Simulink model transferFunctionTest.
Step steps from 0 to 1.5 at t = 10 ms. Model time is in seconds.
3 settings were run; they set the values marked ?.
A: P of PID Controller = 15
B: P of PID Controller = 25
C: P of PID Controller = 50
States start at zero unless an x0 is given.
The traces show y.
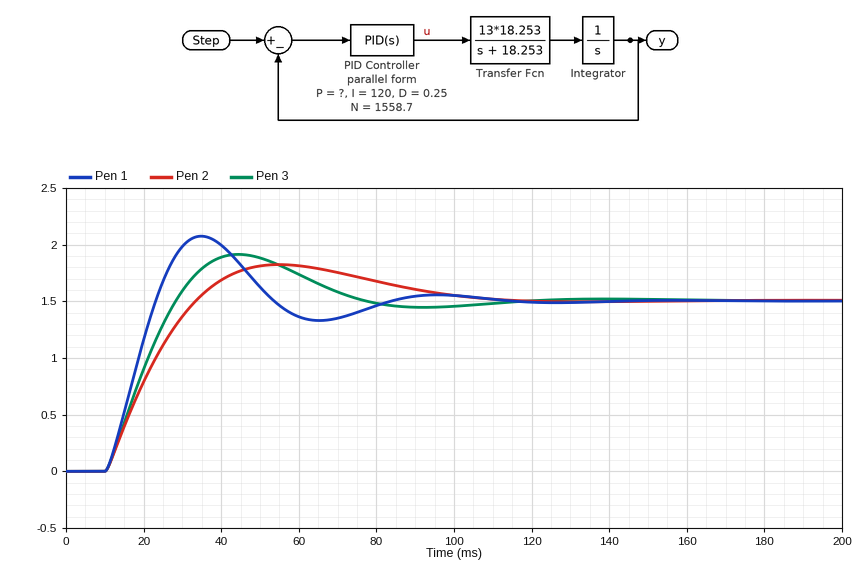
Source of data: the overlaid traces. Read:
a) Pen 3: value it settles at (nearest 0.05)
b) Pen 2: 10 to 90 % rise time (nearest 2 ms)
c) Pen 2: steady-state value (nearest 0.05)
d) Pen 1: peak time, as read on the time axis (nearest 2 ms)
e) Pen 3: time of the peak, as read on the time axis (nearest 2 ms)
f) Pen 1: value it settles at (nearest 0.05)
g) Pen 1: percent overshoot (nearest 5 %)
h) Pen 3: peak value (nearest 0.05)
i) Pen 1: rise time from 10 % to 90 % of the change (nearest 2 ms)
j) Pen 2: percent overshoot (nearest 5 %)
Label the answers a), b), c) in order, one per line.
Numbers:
a) 1.50
b) 18 ms
c) 1.50
d) 34 ms
e) 44 ms
f) 1.50
g) 40 %
h) 1.90
i) 10 ms
j) 20 %
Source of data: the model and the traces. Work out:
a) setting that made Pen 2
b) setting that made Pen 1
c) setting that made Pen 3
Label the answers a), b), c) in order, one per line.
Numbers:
a) A
b) C
c) B
